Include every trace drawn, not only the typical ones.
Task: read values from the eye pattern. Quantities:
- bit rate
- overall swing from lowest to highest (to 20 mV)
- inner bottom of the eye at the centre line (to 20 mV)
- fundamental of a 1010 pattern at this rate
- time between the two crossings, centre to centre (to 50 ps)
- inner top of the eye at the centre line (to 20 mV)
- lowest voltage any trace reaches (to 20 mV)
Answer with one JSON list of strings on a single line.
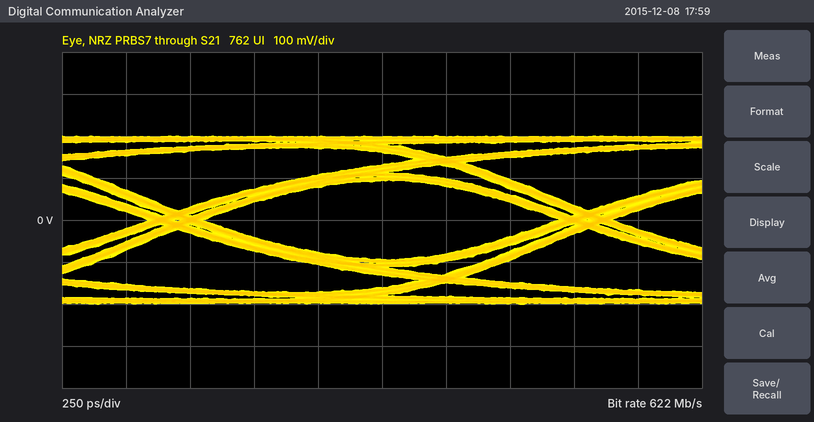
["622 Mb/s", "400 mV", "-100 mV", "311 MHz", "1.60 ns", "100 mV", "-200 mV"]
